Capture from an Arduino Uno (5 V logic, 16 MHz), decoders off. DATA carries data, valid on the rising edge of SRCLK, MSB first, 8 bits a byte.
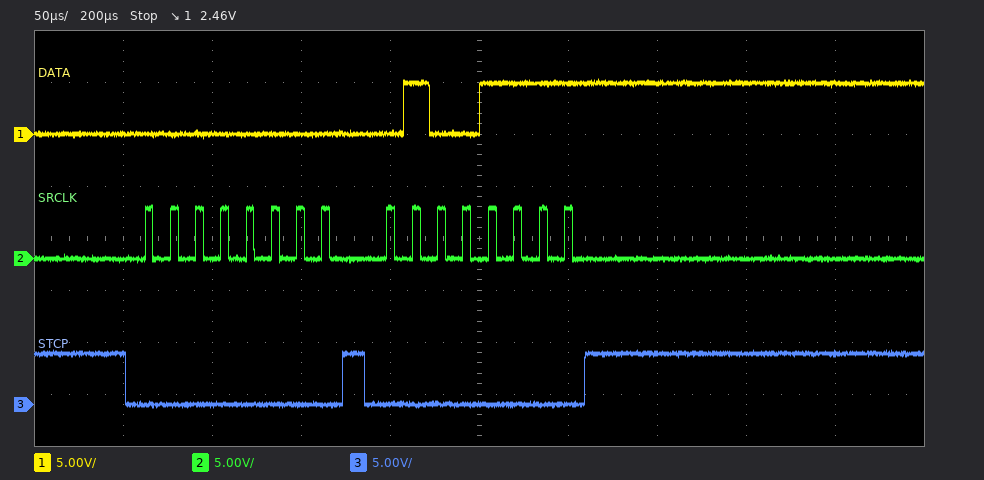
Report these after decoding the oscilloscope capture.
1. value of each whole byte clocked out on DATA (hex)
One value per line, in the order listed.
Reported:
0x00 0x4F
